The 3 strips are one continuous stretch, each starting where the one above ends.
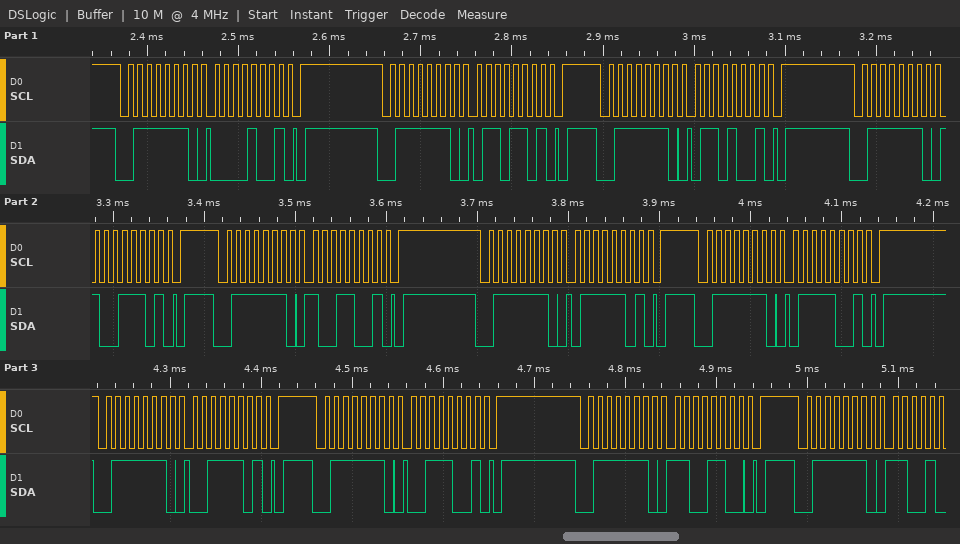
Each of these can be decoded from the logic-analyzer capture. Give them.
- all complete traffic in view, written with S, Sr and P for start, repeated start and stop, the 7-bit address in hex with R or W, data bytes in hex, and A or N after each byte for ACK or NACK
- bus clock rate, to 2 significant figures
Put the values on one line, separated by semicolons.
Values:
S 3FW A 09 A P S 3FW A 6D A P S 3FW A 69 A P S 3FW A 9D A P S 3FW A 99 A P S 3FW A 7D A P S 3FW A 79 A P S 3FW A 3D A P S 3FW A 39 A P S 3FW A CC A P S 3FW A; 100 kHz
